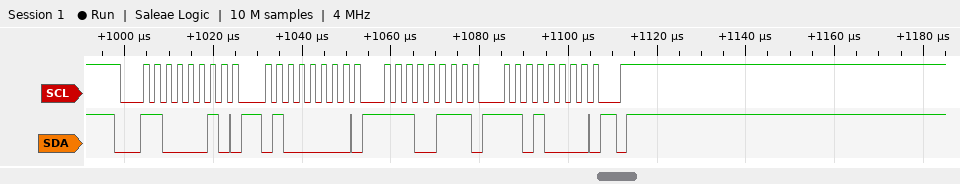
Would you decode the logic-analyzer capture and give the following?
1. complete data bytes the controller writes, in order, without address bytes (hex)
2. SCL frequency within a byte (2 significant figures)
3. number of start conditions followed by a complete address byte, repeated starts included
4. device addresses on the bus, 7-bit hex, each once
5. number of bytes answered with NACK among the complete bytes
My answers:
40 E7 D0
400 kHz
1
0x61
0
